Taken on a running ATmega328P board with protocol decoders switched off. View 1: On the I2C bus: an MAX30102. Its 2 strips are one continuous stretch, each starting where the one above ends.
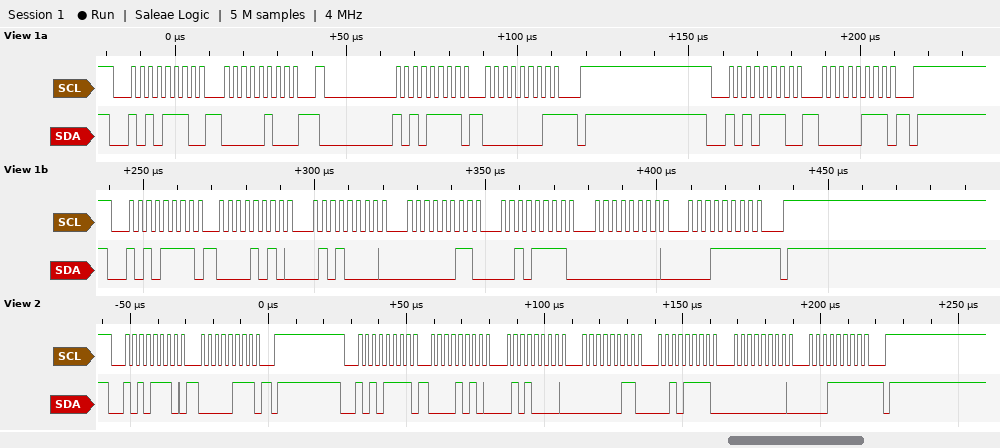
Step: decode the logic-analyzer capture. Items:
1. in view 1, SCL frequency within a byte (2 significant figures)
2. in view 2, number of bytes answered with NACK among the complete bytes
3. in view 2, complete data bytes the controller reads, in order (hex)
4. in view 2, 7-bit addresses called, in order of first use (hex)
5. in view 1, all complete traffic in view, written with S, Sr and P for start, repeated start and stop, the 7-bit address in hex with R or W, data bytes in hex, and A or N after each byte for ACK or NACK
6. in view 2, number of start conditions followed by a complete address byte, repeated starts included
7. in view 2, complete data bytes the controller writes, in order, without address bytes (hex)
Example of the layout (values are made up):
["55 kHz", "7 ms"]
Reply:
["400 kHz", "1", "0A 50 03 2F 00 1F", "0x57", "S 57W A 04 A Sr 57R A 01 N P S 57W A 07 A P S 57R A 0A A 50 A 03 A 2F A 00 A 1F N P", "2", "07"]
